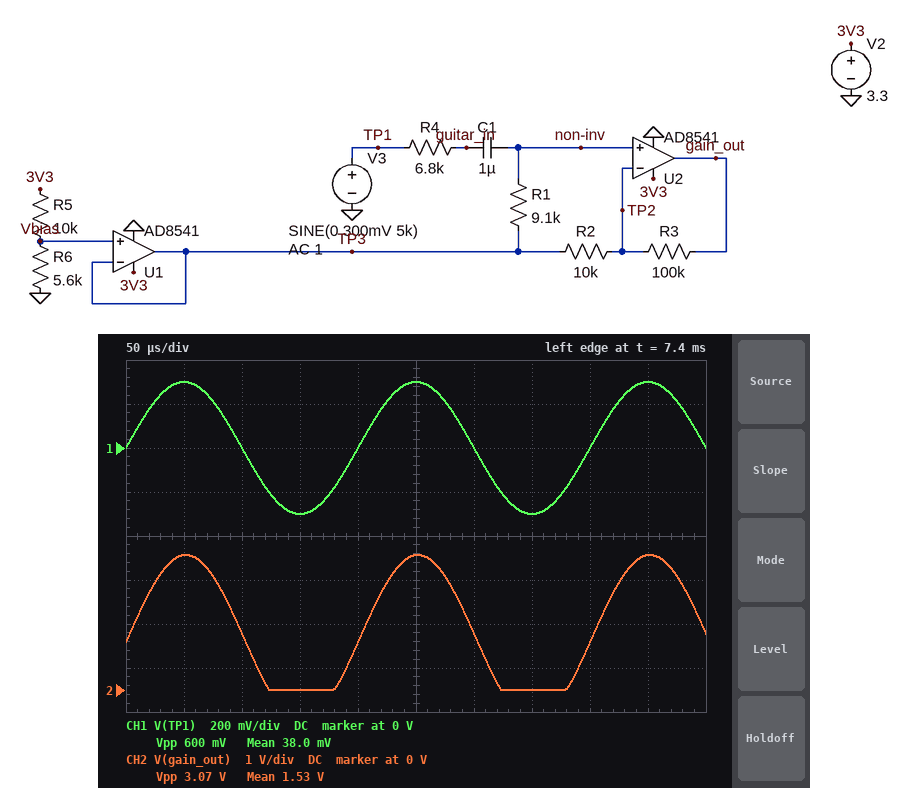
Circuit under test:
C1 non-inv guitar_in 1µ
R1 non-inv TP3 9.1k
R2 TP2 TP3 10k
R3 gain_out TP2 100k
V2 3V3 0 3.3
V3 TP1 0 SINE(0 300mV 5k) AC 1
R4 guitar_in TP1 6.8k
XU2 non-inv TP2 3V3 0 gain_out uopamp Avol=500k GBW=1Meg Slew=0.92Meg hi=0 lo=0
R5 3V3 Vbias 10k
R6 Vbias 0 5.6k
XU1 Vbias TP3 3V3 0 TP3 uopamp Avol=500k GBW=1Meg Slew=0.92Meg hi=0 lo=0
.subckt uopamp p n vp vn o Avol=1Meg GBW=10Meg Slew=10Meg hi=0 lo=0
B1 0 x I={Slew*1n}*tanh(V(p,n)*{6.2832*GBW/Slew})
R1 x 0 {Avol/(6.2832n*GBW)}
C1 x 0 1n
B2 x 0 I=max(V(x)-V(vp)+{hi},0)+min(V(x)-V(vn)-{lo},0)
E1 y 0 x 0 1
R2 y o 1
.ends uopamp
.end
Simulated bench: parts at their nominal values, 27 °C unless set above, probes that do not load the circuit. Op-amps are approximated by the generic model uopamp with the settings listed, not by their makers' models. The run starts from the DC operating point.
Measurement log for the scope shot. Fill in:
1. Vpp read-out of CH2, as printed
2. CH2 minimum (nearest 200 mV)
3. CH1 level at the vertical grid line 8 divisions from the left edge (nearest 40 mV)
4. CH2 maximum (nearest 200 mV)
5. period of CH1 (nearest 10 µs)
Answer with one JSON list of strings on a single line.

["3.07 V", "0 V", "0 V", "3.0 V", "200 µs"]
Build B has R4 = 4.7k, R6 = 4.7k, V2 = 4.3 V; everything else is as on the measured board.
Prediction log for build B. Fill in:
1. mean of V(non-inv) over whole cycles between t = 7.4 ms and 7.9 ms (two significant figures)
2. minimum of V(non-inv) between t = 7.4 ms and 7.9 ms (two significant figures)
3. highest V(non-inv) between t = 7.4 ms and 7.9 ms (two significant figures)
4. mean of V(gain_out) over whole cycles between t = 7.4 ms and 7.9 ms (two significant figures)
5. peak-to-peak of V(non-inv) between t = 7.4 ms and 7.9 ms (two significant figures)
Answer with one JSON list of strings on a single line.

["1.4 V", "1.2 V", "1.6 V", "1.5 V", "400 mV"]
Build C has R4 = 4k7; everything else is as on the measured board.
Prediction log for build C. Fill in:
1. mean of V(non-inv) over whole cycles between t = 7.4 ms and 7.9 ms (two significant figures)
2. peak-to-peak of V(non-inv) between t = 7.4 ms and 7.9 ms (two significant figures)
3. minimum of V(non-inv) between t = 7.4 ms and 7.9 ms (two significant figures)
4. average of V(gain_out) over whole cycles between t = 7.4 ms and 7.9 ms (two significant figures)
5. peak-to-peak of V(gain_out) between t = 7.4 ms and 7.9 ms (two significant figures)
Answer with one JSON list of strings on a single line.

["1.2 V", "400 mV", "990 mV", "1.4 V", "3.3 V"]
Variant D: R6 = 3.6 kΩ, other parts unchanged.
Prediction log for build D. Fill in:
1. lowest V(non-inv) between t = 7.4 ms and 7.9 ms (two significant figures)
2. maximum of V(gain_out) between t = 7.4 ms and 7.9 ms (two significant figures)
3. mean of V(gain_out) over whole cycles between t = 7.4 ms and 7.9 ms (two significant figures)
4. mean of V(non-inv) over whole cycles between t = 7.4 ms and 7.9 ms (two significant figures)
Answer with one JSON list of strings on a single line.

["700 mV", "2.8 V", "1.1 V", "870 mV"]
